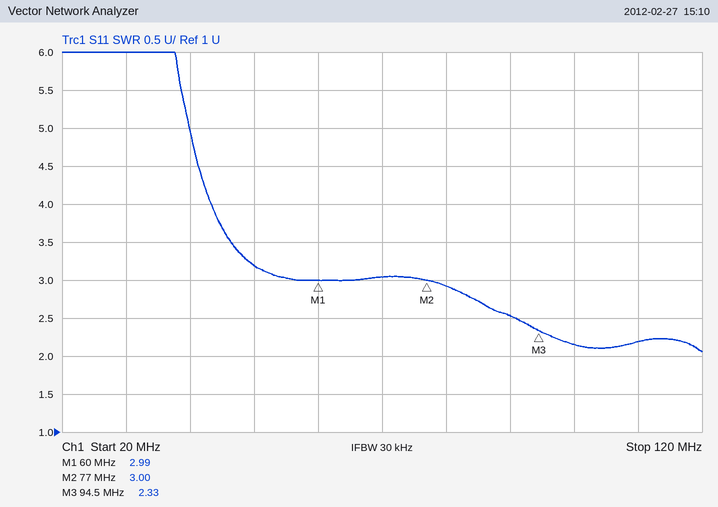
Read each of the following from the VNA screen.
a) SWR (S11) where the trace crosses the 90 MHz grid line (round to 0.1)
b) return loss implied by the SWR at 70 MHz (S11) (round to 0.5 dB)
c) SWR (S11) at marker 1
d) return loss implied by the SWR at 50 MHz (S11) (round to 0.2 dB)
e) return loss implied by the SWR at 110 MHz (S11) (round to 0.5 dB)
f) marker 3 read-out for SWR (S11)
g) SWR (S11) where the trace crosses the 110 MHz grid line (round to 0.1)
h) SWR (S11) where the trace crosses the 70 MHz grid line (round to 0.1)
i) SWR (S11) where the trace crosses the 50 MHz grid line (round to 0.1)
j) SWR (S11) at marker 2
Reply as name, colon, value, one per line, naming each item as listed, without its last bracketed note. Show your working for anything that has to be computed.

SWR (S11) where the trace crosses the 90 MHz grid line: 2.5
return loss implied by the SWR at 70 MHz (S11): −20 log10((3 − 1)/(3 + 1)) ≈ 6.0 dB
SWR (S11) at marker 1: 2.99
return loss implied by the SWR at 50 MHz (S11): −20 log10((3.2 − 1)/(3.2 + 1)) ≈ 5.6 dB
return loss implied by the SWR at 110 MHz (S11): −20 log10((2.2 − 1)/(2.2 + 1)) ≈ 8.5 dB
marker 3 read-out for SWR: 2.33
SWR (S11) where the trace crosses the 110 MHz grid line: 2.2
SWR (S11) where the trace crosses the 70 MHz grid line: 3.0
SWR (S11) where the trace crosses the 50 MHz grid line: 3.2
SWR (S11) at marker 2: 3.00
